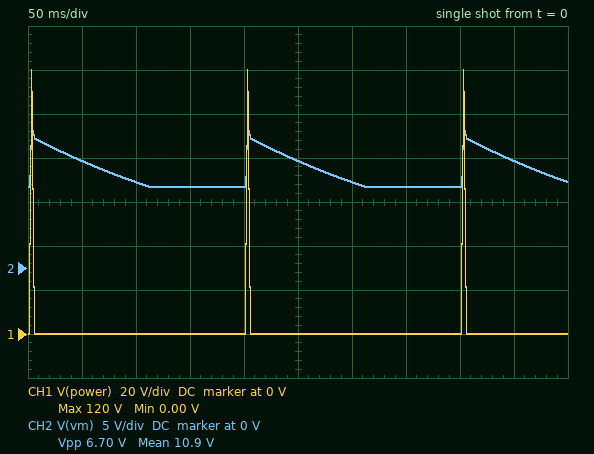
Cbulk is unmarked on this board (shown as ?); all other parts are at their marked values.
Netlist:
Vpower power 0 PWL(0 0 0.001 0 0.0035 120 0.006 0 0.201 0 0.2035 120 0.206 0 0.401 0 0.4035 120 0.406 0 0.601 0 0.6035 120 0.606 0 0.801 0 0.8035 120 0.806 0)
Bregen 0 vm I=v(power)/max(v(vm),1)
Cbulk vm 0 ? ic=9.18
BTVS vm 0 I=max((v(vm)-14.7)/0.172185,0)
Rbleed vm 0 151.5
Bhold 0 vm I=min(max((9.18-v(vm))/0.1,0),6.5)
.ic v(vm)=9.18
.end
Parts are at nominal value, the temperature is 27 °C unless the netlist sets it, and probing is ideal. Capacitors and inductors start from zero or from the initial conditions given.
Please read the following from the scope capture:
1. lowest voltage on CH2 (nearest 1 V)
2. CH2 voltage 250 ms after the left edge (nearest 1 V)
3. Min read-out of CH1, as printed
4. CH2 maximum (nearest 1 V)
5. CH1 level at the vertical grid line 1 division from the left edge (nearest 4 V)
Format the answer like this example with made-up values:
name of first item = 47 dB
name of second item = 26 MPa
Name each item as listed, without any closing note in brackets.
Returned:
lowest voltage on CH2 = 9 V
CH2 voltage 250 ms after the left edge = 12 V
Min read-out of CH1, as printed = 0.00 V
CH2 maximum = 16 V
CH1 level at the vertical grid line 1 division from the left edge = 0 V
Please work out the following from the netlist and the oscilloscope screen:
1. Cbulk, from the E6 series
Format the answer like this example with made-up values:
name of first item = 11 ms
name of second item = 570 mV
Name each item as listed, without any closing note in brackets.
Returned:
Cbulk, from the E6 series = 1.5 mF
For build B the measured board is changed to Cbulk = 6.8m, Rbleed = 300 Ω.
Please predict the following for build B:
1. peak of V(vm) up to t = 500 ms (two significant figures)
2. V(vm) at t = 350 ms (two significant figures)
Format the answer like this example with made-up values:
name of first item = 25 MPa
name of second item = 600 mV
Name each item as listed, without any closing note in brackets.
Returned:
peak of V(vm) up to t = 500 ms = 15 V
V(vm) at t = 350 ms = 14 V
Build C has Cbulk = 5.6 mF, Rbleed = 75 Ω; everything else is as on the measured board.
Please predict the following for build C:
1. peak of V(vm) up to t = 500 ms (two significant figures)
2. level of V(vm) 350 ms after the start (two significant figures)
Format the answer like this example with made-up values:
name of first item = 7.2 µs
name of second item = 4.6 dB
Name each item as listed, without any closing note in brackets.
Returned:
peak of V(vm) up to t = 500 ms = 14 V
level of V(vm) 350 ms after the start = 9.7 V
